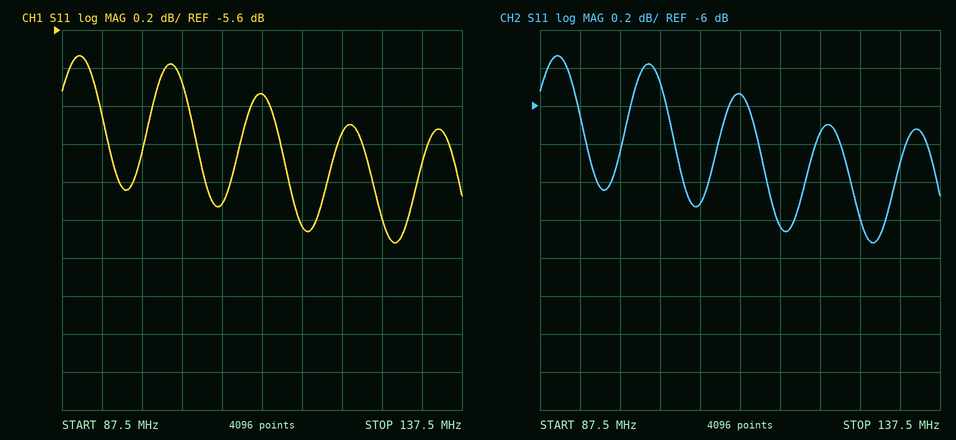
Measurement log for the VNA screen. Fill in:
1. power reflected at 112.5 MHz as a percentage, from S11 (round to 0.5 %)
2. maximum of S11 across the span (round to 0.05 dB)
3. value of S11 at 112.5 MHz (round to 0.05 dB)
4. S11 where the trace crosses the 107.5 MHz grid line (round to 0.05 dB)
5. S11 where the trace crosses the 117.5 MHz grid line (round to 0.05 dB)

25.5 %
-5.75 dB
-5.95 dB
-6.50 dB
-6.65 dB
